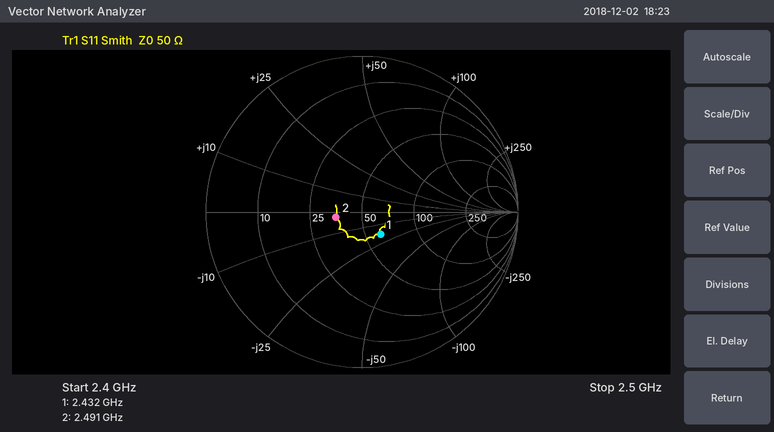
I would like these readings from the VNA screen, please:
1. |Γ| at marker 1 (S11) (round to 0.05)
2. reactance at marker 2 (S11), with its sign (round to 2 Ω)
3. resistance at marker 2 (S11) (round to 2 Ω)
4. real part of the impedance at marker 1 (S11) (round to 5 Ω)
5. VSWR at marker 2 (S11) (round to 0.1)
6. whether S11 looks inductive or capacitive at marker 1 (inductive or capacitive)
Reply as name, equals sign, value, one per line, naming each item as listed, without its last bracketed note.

|Γ| at marker 1 (S11) = 0.20
reactance at marker 2 (S11), with its sign = -2 Ω
resistance at marker 2 (S11) = 36 Ω
real part of the impedance at marker 1 (S11) = 60 Ω
VSWR at marker 2 (S11) = 1.4
whether S11 looks inductive or capacitive at marker 1 = capacitive
